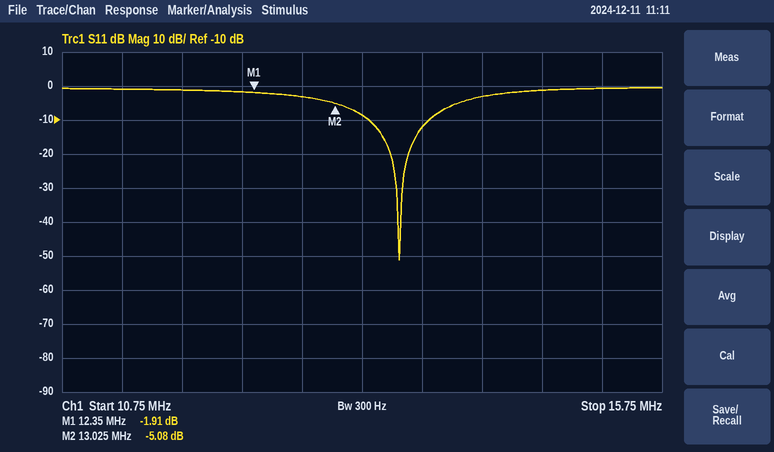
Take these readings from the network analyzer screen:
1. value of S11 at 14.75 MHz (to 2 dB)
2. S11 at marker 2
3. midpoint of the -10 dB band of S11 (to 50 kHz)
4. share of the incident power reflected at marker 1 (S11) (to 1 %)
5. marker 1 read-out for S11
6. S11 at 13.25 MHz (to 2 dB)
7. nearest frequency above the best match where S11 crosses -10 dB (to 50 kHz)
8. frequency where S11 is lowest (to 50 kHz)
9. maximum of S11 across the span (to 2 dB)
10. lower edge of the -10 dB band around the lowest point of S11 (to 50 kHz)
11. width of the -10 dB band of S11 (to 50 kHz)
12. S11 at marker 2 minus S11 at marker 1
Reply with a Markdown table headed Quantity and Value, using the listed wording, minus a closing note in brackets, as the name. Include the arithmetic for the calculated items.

| Quantity | Value |
|---|---|
| value of S11 at 14.75 MHz | -2 dB |
| S11 at marker 2 | -5.08 dB |
| midpoint of the -10 dB band of S11 | 13.55 MHz |
| share of the incident power reflected at marker 1 (S11) | 10^(-1.91/10) ≈ 64 % |
| marker 1 read-out for S11 | -1.91 dB |
| S11 at 13.25 MHz | -8 dB |
| nearest frequency above the best match where S11 crosses -10 dB | 13.80 MHz |
| frequency where S11 is lowest | 13.55 MHz |
| maximum of S11 across the span | 0 dB |
| lower edge of the -10 dB band around the lowest point of S11 | 13.30 MHz |
| width of the -10 dB band of S11 | 13.80 MHz − 13.30 MHz = 500 kHz |
| S11 at marker 2 minus S11 at marker 1 | -5.08 − (-1.91) = -3.17 dB |
